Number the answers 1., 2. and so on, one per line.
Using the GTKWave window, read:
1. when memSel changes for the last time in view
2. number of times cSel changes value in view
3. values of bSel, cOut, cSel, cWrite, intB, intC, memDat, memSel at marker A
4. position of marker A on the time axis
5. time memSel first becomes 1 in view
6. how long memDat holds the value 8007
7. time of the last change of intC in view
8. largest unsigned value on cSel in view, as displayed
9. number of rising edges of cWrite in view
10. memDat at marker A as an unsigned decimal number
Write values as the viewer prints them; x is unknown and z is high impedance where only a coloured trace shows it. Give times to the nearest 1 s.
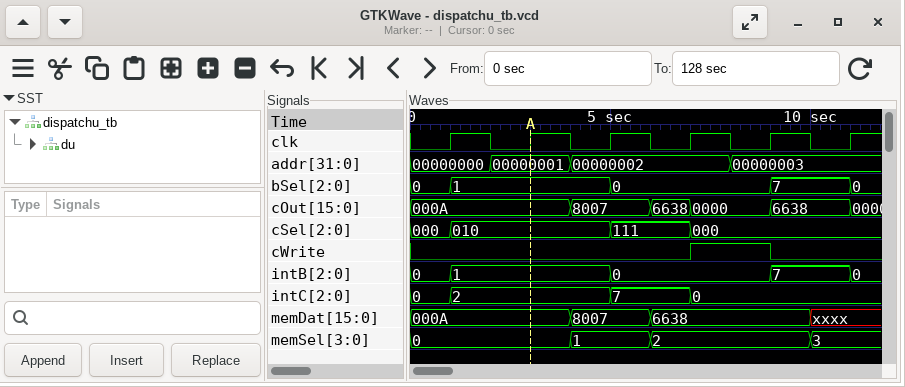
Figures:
1. 10 s
2. 3
3. bSel=1, cOut=000A, cSel=010, cWrite=0, intB=1, intC=2, memDat=000A, memSel=0
4. 3 s
5. 4 s
6. 2 s
7. 7 s
8. 111
9. 1
10. 10
